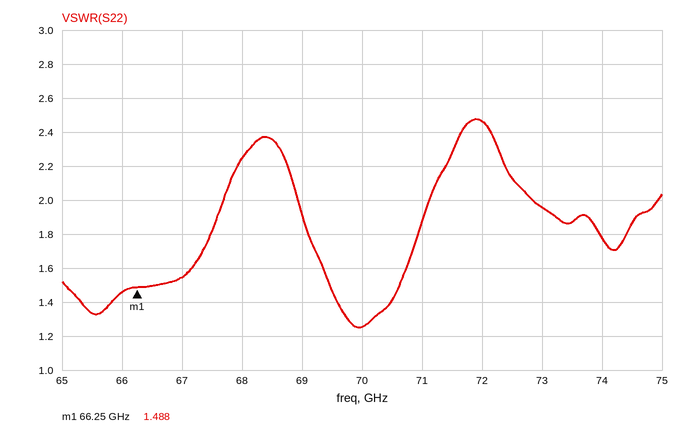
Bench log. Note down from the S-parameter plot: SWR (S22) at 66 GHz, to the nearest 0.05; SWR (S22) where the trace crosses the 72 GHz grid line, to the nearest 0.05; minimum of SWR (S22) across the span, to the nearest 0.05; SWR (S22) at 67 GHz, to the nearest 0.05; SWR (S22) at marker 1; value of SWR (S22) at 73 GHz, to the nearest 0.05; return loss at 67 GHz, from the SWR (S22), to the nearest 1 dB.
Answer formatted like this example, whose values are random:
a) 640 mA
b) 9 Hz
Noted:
a) 1.45
b) 2.45
c) 1.25
d) 1.55
e) 1.488
f) 1.95
g) 13 dB
